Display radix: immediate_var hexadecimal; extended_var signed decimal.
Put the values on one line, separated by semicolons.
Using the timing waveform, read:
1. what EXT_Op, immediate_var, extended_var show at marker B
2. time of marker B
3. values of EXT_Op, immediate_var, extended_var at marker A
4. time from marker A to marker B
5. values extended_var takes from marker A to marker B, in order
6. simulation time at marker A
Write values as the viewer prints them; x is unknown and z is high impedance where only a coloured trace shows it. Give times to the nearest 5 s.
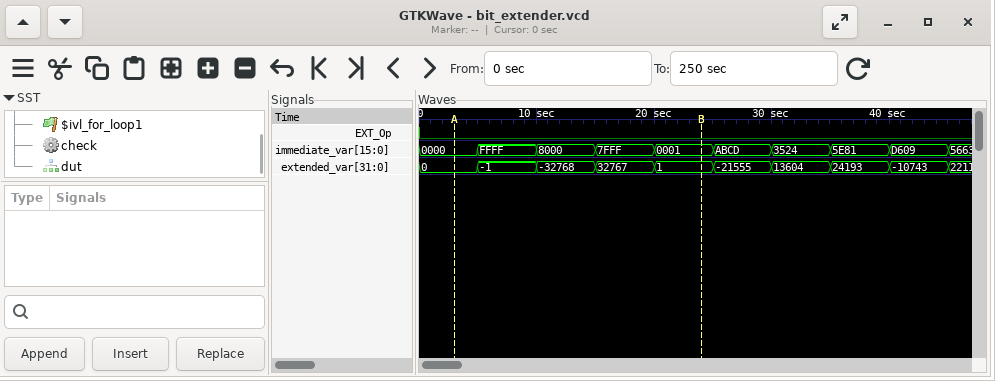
EXT_Op=0, immediate_var=0001, extended_var=1; 25 s; EXT_Op=0, immediate_var=0000, extended_var=0; 20 s; 0, -1, -32768, 32767, 1; 5 s
